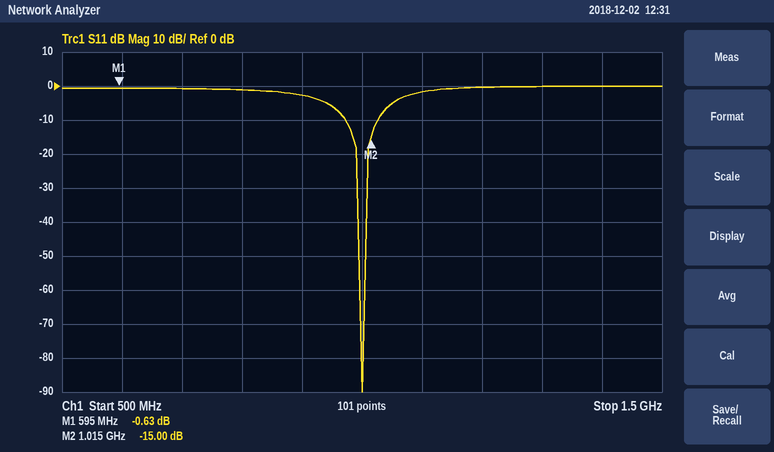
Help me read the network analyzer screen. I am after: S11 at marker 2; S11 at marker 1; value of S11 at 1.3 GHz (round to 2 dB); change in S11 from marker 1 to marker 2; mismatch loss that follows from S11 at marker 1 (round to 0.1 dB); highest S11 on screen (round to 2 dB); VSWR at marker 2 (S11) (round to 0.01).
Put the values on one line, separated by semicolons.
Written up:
-15.00 dB; -0.63 dB; 0 dB; -14.37 dB; 8.7 dB; 0 dB; 1.43
